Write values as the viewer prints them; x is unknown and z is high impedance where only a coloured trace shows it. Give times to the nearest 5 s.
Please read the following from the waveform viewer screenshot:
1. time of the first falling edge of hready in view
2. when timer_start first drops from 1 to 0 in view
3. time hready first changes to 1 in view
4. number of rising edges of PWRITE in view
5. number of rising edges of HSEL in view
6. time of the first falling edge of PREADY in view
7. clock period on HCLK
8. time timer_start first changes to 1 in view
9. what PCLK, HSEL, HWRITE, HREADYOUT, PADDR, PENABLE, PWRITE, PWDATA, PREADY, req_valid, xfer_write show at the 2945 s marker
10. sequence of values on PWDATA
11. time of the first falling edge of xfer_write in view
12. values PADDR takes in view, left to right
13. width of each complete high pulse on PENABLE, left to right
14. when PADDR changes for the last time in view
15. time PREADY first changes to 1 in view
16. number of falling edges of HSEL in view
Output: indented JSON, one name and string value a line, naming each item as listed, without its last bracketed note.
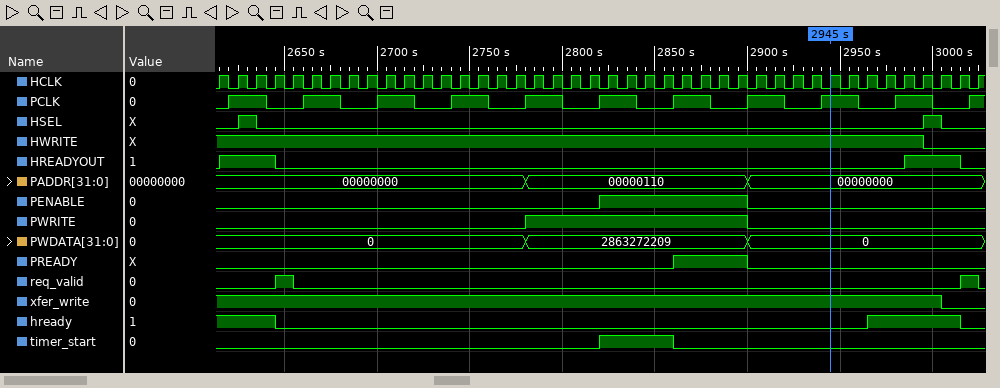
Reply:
{
  "time of the first falling edge of hready in view": "2645 s",
  "when timer_start first drops from 1 to 0 in view": "2860 s",
  "time hready first changes to 1 in view": "2965 s",
  "number of rising edges of PWRITE in view": "1",
  "number of rising edges of HSEL in view": "2",
  "time of the first falling edge of PREADY in view": "2900 s",
  "clock period on HCLK": "10 s",
  "time timer_start first changes to 1 in view": "2820 s",
  "what PCLK, HSEL, HWRITE, HREADYOUT, PADDR, PENABLE, PWRITE, PWDATA, PREADY, req_valid, xfer_write show at the 2945 s marker": "PCLK=1, HSEL=0, HWRITE=1, HREADYOUT=0, PADDR=00000000, PENABLE=0, PWRITE=0, PWDATA=0, PREADY=0, req_valid=0, xfer_write=1",
  "sequence of values on PWDATA": "0, 2863272209, 0",
  "time of the first falling edge of xfer_write in view": "3005 s",
  "values PADDR takes in view, left to right": "00000000, 00000110, 00000000",
  "width of each complete high pulse on PENABLE, left to right": "80 s",
  "when PADDR changes for the last time in view": "2900 s",
  "time PREADY first changes to 1 in view": "2860 s",
  "number of falling edges of HSEL in view": "2"
}
